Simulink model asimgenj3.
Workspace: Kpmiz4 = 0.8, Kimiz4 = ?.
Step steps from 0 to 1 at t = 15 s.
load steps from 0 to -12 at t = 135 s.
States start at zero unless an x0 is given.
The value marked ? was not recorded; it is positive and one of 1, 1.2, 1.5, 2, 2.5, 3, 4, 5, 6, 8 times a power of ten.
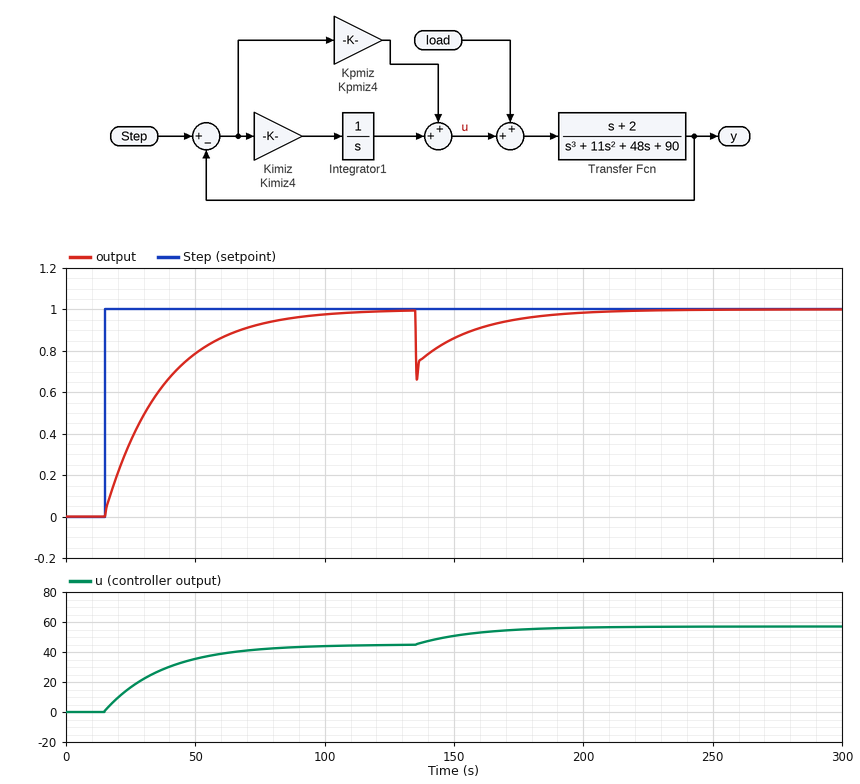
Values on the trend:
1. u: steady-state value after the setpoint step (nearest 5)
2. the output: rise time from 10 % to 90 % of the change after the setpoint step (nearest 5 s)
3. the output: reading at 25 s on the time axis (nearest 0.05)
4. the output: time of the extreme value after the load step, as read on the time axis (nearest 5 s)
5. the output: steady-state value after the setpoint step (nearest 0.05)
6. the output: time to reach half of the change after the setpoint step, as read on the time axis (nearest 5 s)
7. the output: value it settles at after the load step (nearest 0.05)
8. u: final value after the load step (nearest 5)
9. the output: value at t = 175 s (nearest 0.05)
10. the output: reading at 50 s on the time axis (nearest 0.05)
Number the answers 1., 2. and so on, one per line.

1. 45
2. 50 s
3. 0.35
4. 135 s
5. 1.00
6. 30 s
7. 1.00
8. 55
9. 0.95
10. 0.80
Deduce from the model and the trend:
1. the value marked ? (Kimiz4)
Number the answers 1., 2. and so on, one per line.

1. 2
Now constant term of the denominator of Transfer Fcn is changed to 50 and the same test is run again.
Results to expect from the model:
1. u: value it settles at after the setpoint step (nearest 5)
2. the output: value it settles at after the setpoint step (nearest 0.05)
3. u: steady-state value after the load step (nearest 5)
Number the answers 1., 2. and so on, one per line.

1. 25
2. 1.00
3. 35
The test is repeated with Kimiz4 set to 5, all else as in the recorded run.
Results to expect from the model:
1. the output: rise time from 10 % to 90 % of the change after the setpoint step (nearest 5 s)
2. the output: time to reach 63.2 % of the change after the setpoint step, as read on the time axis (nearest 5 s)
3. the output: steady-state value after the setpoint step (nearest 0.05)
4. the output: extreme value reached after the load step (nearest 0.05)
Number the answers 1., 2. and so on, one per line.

1. 20 s
2. 25 s
3. 1.00
4. 0.65
